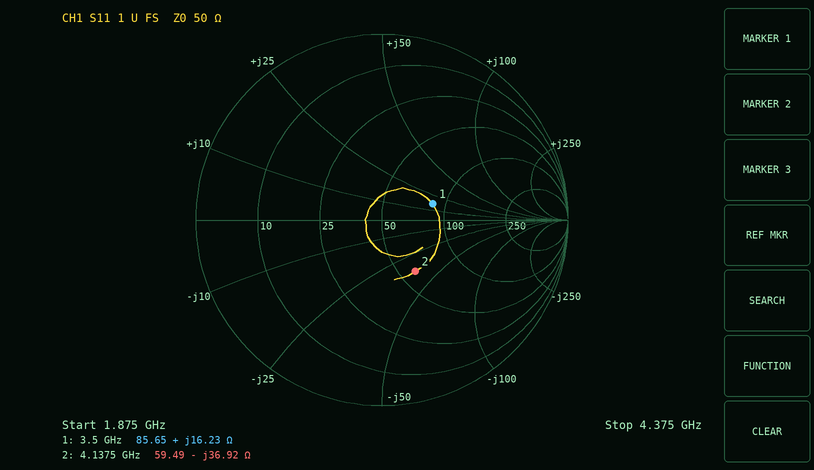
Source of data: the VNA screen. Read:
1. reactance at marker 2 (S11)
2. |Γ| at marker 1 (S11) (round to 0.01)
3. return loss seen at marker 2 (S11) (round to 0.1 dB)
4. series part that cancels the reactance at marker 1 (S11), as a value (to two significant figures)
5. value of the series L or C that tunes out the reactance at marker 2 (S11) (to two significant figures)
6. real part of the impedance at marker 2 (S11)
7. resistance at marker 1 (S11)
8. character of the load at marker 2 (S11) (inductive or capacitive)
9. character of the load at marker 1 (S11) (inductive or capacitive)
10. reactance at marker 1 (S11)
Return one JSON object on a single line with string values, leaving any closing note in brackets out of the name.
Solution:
{"reactance at marker 2": "-36.92 Ω", "|Γ| at marker 1 (S11)": "0.29", "return loss seen at marker 2 (S11)": "9.6 dB", "series part that cancels the reactance at marker 1 (S11), as a value": "2.8 pF", "value of the series L or C that tunes out the reactance at marker 2 (S11)": "1.4 nH", "real part of the impedance at marker 2": "59.49 Ω", "resistance at marker 1": "85.65 Ω", "character of the load at marker 2 (S11)": "capacitive", "character of the load at marker 1 (S11)": "inductive", "reactance at marker 1": "+16.23 Ω"}
